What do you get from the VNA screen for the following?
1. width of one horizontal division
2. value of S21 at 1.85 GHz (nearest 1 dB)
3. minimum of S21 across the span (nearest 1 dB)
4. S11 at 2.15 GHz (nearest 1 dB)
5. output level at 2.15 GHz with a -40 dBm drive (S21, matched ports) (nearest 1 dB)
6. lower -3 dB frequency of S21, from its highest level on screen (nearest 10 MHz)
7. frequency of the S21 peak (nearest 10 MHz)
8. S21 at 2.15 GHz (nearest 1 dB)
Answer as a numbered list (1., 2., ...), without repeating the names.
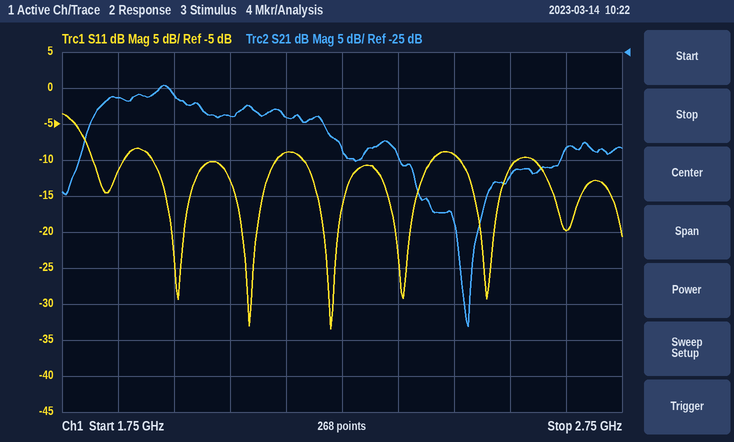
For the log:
1. 100 MHz
2. -31 dB
3. -63 dB
4. -9 dB
5. -74 dBm
6. 1.82 GHz
7. 1.93 GHz
8. -34 dB
